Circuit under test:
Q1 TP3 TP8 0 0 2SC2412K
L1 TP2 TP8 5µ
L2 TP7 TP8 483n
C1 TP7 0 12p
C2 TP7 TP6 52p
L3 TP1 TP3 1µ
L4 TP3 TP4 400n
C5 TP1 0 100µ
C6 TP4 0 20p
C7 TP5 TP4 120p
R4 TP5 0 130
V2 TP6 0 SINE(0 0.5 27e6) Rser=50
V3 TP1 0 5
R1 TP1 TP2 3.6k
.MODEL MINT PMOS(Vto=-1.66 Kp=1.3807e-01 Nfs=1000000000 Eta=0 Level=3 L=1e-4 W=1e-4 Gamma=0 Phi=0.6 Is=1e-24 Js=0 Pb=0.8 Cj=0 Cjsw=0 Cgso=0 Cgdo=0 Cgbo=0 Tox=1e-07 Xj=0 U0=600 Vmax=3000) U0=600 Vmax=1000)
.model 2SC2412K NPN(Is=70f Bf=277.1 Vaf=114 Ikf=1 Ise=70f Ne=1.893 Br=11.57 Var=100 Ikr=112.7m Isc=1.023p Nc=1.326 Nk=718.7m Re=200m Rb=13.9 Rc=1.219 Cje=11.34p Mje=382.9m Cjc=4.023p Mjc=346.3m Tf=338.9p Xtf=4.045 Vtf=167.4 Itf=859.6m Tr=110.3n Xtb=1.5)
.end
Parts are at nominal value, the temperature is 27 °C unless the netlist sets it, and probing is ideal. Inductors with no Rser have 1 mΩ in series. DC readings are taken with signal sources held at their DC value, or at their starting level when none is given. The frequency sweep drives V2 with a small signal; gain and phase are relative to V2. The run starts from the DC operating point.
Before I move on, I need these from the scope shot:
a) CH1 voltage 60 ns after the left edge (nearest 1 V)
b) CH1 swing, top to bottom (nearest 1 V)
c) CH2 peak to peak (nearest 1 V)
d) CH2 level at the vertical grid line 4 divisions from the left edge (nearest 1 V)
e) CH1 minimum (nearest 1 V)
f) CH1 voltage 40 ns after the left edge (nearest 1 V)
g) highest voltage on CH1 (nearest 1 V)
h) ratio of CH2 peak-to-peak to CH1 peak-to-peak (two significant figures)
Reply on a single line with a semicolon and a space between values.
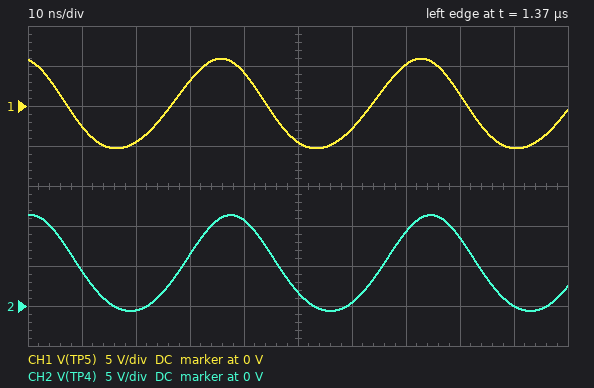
-3 V; 11 V; 12 V; 11 V; -5 V; 4 V; 6 V; 1.1
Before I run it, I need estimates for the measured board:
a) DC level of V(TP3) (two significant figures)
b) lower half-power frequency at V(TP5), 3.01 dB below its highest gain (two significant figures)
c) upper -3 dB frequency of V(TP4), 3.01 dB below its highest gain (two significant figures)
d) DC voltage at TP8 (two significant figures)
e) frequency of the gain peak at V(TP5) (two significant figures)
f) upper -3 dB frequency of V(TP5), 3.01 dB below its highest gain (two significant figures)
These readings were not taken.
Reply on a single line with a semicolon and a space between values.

5.0 V; 16 MHz; 34 MHz; 820 mV; 27 MHz; 34 MHz
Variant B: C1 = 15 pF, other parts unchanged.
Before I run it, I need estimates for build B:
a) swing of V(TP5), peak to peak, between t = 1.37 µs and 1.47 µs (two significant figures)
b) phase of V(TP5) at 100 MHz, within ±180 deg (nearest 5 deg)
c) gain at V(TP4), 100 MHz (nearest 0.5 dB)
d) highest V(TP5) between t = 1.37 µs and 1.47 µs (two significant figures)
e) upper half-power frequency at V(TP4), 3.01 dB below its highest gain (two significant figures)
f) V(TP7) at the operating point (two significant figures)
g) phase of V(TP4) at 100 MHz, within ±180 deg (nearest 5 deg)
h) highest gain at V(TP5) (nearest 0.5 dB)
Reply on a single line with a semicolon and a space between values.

12 V; -100 deg; -10.5 dB; 6.1 V; 33 MHz; 820 mV; -105 deg; 21.5 dB
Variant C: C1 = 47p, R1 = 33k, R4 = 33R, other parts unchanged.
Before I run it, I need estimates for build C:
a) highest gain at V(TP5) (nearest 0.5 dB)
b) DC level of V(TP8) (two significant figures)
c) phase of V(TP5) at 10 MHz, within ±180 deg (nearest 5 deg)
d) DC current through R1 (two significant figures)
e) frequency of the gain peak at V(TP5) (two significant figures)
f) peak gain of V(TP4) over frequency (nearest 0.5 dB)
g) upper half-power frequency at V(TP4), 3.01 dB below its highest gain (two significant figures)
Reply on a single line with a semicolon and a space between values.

17.5 dB; 710 mV; -80 deg; 130 µA; 25 MHz; 26.5 dB; 15 MHz
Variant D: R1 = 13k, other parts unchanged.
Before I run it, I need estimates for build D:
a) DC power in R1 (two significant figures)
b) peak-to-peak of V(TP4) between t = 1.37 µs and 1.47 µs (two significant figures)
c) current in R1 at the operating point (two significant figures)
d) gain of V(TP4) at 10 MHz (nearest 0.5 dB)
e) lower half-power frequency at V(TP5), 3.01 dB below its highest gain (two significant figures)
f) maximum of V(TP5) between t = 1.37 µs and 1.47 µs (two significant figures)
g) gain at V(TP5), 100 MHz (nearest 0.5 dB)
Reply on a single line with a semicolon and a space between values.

1.4 mW; 15 V; 330 µA; 21.0 dB; 17 MHz; 7.8 V; -6.5 dB
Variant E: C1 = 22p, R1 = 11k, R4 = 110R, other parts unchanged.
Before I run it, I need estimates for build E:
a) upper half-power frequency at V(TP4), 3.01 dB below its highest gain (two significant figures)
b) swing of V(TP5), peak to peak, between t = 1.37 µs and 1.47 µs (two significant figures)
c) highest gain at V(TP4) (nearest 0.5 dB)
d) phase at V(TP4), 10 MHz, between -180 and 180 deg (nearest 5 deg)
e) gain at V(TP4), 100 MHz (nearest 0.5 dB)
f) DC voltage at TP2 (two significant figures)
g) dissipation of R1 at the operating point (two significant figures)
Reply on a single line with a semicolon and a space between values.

32 MHz; 14 V; 25.0 dB; -150 deg; -9.0 dB; 750 mV; 1.6 mW
